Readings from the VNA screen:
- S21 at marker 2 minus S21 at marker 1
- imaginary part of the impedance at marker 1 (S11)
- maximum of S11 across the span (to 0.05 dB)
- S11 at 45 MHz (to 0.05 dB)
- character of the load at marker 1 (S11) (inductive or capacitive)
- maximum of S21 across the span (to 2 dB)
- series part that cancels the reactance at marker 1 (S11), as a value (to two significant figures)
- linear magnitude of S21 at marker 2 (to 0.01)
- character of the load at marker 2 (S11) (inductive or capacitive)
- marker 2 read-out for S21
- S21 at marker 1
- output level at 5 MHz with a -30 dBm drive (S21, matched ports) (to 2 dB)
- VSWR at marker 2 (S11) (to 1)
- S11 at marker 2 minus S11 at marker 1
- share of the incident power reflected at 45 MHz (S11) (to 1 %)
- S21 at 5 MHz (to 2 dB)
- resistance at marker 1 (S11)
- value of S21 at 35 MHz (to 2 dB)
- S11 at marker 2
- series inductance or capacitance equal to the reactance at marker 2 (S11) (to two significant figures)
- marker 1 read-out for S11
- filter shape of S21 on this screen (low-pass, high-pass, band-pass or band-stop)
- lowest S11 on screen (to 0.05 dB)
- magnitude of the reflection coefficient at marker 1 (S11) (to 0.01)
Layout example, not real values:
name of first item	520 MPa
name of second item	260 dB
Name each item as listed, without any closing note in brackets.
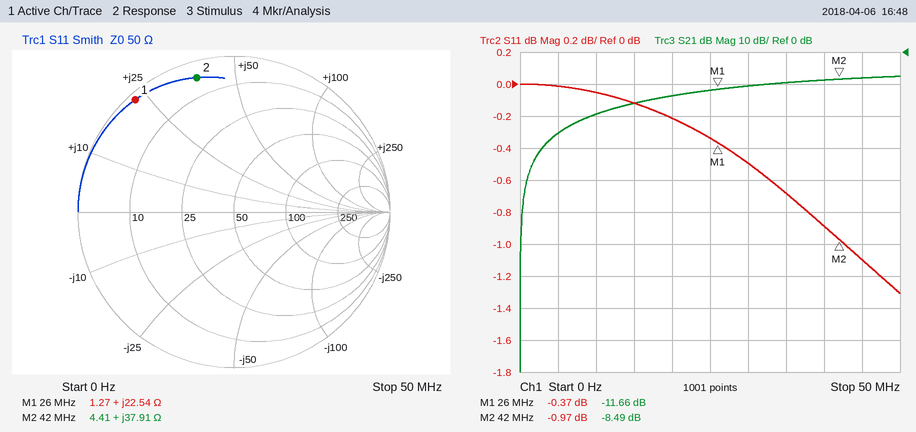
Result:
S21 at marker 2 minus S21 at marker 1	3.17 dB
imaginary part of the impedance at marker 1	+22.54 Ω
maximum of S11 across the span	0.00 dB
S11 at 45 MHz	-1.10 dB
character of the load at marker 1 (S11)	inductive
maximum of S21 across the span	-8 dB
series part that cancels the reactance at marker 1 (S11), as a value	270 pF
linear magnitude of S21 at marker 2	0.38
character of the load at marker 2 (S11)	inductive
marker 2 read-out for S21	-8.49 dB
S21 at marker 1	-11.66 dB
output level at 5 MHz with a -30 dBm drive (S21, matched ports)	-56 dBm
VSWR at marker 2 (S11)	18
S11 at marker 2 minus S11 at marker 1	-0.60 dB
share of the incident power reflected at 45 MHz (S11)	78 %
S21 at 5 MHz	-26 dB
resistance at marker 1	1.27 Ω
value of S21 at 35 MHz	-10 dB
S11 at marker 2	-0.97 dB
series inductance or capacitance equal to the reactance at marker 2 (S11)	140 nH
marker 1 read-out for S11	-0.37 dB
filter shape of S21 on this screen	high-pass
lowest S11 on screen	-1.30 dB
magnitude of the reflection coefficient at marker 1 (S11)	0.96
